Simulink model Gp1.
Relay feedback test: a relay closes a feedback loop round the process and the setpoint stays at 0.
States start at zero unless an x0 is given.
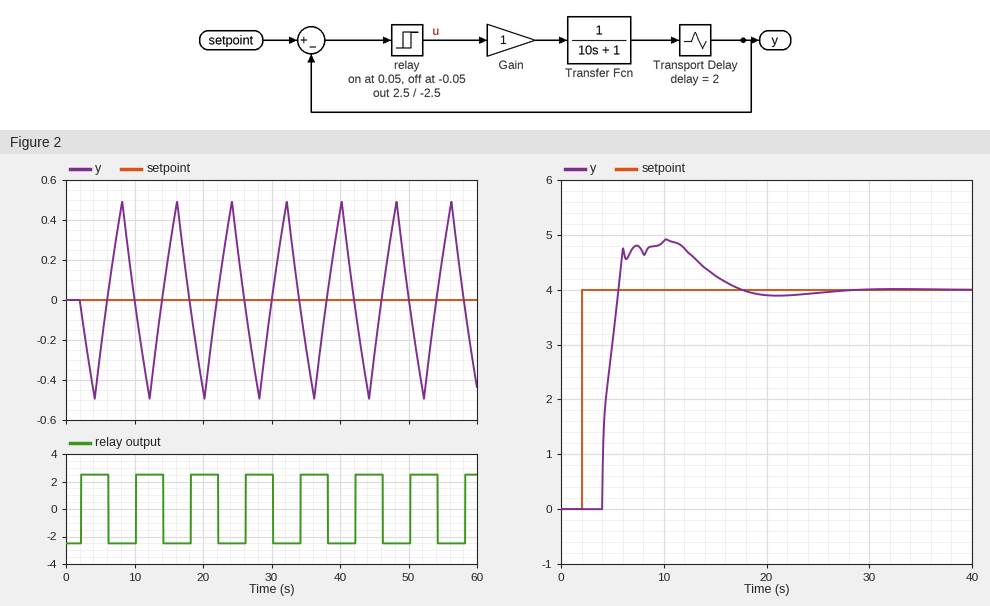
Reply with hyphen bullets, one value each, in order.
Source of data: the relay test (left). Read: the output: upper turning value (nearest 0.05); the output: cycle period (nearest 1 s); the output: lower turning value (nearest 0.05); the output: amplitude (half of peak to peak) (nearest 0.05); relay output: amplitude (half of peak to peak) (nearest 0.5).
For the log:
- 0.50
- 8 s
- -0.50
- 0.50
- 2.5
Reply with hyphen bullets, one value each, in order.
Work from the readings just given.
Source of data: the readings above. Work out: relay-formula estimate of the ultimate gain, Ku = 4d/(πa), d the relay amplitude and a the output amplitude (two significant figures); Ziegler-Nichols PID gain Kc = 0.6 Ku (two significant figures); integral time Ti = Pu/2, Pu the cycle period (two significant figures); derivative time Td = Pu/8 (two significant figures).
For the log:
- 6.4
- 3.8
- 4.0 s
- 1.0 s
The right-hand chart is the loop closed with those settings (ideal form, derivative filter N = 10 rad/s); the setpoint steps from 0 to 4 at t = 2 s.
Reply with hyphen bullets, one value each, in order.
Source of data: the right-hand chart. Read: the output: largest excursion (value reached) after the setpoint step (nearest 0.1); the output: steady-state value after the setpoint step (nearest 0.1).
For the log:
- 4.9
- 4.0
